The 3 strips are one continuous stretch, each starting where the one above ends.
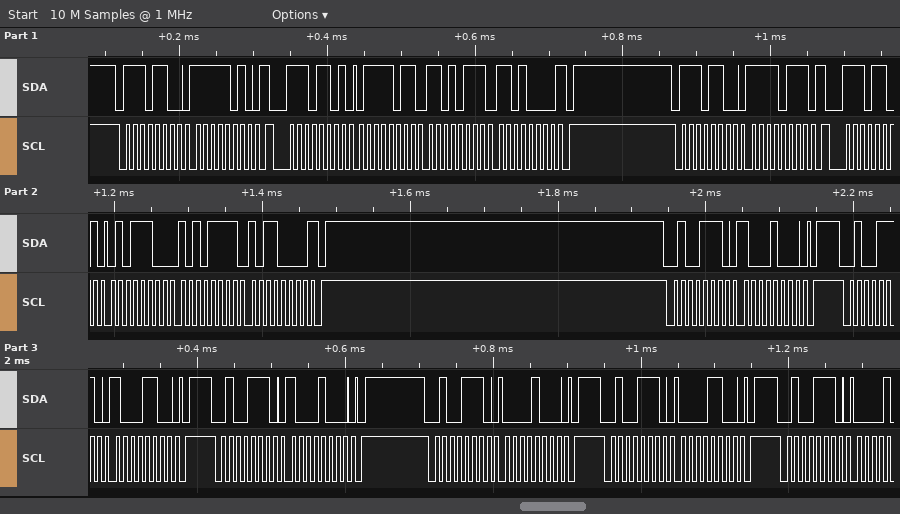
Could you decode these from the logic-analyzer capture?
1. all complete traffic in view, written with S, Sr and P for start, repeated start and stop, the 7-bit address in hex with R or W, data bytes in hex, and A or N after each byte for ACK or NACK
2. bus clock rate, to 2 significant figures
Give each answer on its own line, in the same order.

S 76W A FA A Sr 76R A 7B A D7 A D0 N P S 76W A F7 A Sr 76R A 5C A AF A B0 N P S 27W A 88 A P S 27W A 8C A P S 27W A 88 A P S 27W A 08 A P S 27W A 0C A P S 27W A
100 kHz
